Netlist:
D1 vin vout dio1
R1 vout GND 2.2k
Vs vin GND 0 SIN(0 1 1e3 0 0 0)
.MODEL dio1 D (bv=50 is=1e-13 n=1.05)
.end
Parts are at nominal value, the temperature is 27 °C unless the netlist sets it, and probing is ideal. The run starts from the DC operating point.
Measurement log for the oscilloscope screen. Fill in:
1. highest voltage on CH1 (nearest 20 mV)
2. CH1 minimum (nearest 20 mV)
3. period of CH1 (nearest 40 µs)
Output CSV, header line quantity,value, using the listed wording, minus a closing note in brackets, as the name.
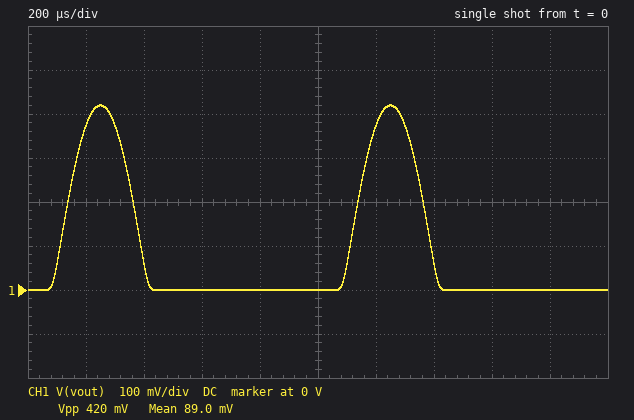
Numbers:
quantity,value
highest voltage on CH1,420 mV
CH1 minimum,0 V
period of CH1,1.00 ms
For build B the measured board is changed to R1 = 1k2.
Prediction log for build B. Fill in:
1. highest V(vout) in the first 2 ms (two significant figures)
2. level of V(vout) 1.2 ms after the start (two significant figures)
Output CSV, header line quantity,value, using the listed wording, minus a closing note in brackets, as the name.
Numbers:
quantity,value
highest V(vout) in the first 2 ms,400 mV
level of V(vout) 1.2 ms after the start,360 mV
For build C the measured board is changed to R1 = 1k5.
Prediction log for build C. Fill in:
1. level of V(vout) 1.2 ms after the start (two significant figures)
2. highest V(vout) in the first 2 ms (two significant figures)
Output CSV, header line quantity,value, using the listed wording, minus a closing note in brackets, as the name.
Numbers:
quantity,value
level of V(vout) 1.2 ms after the start,360 mV
highest V(vout) in the first 2 ms,410 mV
